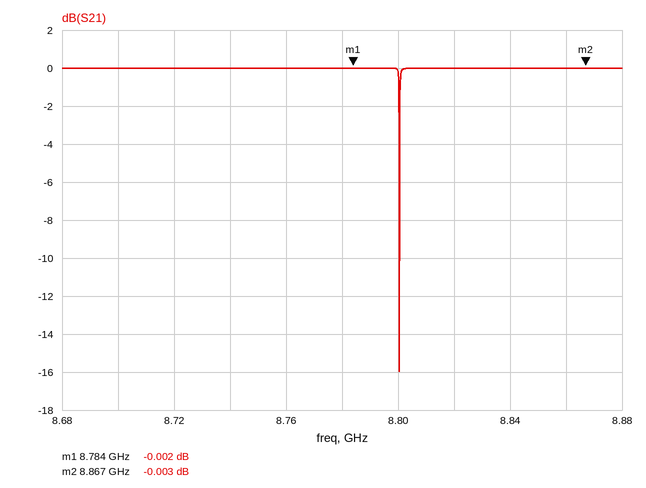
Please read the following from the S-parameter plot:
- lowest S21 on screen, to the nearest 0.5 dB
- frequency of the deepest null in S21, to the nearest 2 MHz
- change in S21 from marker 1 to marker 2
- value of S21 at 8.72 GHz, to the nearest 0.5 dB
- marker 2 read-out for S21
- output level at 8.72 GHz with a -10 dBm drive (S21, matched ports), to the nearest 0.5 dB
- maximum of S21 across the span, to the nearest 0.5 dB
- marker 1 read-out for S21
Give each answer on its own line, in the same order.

-16.0 dB
8.800 GHz
-0.001 dB
0.0 dB
-0.003 dB
-10.0 dBm
0.0 dB
-0.002 dB
